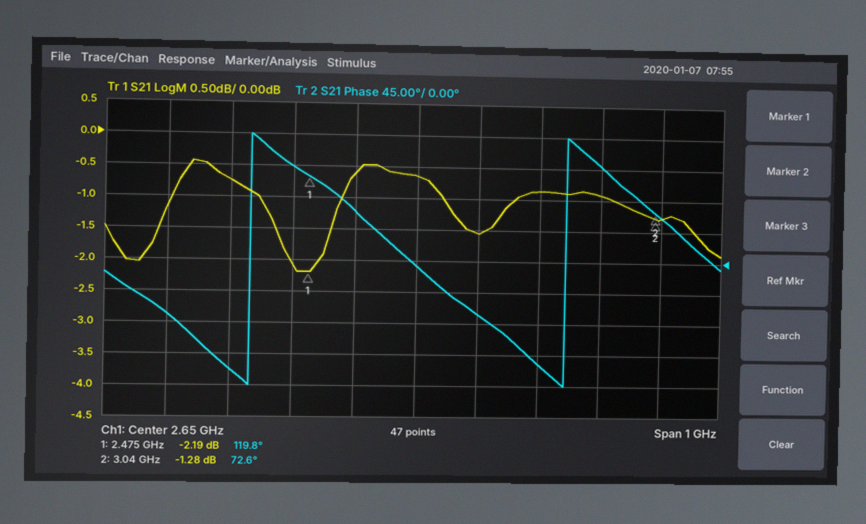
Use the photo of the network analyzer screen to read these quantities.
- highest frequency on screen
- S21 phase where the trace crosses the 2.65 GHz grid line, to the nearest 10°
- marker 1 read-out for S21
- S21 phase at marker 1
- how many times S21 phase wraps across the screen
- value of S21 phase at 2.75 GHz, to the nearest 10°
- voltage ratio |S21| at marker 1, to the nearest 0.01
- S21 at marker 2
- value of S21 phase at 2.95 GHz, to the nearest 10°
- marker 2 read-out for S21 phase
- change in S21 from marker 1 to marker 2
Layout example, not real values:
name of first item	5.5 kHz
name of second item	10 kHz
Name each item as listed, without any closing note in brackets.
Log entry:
highest frequency on screen	3.15 GHz
S21 phase where the trace crosses the 2.65 GHz grid line, to the nearest 10°	-10°
marker 1 read-out for S21	-2.19 dB
S21 phase at marker 1	119.8°
how many times S21 phase wraps across the screen	2
value of S21 phase at 2.75 GHz, to the nearest 10°	-80°
voltage ratio |S21| at marker 1, to the nearest 0.01	0.78
S21 at marker 2	-1.28 dB
value of S21 phase at 2.95 GHz, to the nearest 10°	140°
marker 2 read-out for S21 phase	72.6°
change in S21 from marker 1 to marker 2	0.91 dB
